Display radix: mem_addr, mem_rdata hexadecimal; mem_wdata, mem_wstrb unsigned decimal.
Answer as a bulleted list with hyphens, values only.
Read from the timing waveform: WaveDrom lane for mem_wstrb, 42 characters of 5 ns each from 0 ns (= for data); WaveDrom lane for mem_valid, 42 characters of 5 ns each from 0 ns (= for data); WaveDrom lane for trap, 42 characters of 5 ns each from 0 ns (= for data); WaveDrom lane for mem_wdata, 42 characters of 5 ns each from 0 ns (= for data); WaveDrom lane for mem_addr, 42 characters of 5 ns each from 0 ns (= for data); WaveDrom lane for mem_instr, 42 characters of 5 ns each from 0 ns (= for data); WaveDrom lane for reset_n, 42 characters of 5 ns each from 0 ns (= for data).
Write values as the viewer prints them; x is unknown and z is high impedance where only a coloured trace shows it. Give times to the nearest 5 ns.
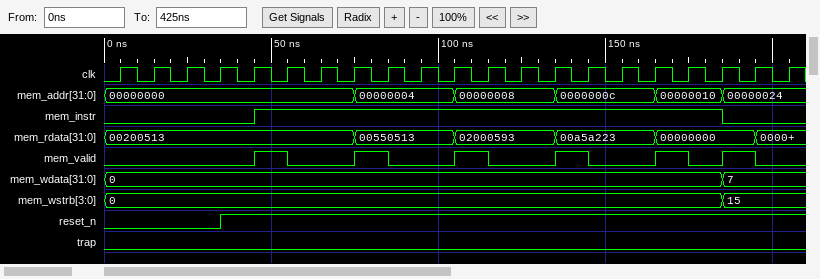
- {name: 'mem_wstrb', wave: '=....................................=....', data: '0 15'}
- {name: 'mem_valid', wave: '0........1.0...1.0...1.0...1.0...1.0.1.0..'}
- {name: 'trap', wave: '0.........................................'}
- {name: 'mem_wdata', wave: '=....................................=....', data: '0 7'}
- {name: 'mem_addr', wave: '=..............=.....=.....=.....=...=....', data: '00000000 00000004 00000008 0000000c 00000010 00000024'}
- {name: 'mem_instr', wave: '0........1...........................0....'}
- {name: 'reset_n', wave: '0......1..................................'}
